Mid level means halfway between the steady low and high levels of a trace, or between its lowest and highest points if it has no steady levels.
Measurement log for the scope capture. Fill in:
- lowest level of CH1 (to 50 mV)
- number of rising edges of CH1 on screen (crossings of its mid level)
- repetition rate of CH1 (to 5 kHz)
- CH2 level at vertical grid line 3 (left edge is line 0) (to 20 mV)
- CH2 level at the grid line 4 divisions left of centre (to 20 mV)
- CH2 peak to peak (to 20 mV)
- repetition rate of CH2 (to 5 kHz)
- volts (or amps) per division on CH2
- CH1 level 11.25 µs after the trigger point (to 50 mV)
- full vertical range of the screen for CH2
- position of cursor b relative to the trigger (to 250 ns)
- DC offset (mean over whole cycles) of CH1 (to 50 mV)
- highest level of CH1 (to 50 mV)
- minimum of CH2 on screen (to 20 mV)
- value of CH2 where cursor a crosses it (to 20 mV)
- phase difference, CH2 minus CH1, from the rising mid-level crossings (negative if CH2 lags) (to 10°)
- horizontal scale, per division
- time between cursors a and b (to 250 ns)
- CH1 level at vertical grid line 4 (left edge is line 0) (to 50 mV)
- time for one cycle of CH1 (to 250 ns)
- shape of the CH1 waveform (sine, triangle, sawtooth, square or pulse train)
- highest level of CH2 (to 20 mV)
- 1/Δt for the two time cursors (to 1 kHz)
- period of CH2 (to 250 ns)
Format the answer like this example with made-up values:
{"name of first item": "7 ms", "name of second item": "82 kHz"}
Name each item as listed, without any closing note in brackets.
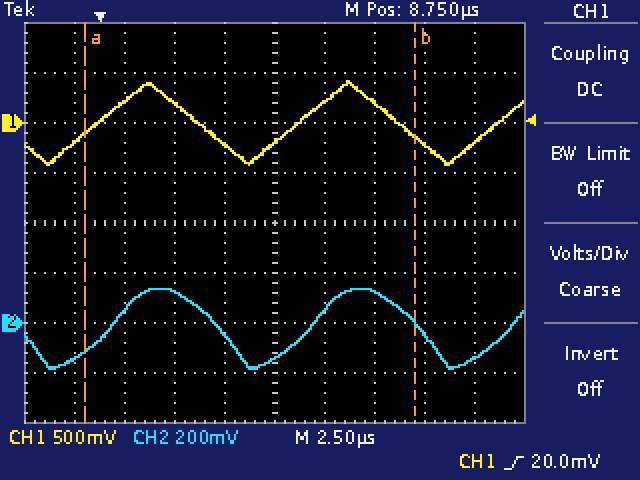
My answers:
{"lowest level of CH1": "-400 mV", "number of rising edges of CH1 on screen": "3", "repetition rate of CH1": "100 kHz", "CH2 level at vertical grid line 3 (left edge is line 0)": "120 mV", "CH2 level at the grid line 4 divisions left of centre": "-140 mV", "CH2 peak to peak": "320 mV", "repetition rate of CH2": "100 kHz", "volts (or amps) per division on CH2": "200 mV", "CH1 level 11.25 µs after the trigger point": "200 mV", "full vertical range of the screen for CH2": "1.6 V", "position of cursor b relative to the trigger": "+15.75 µs", "DC offset (mean over whole cycles) of CH1": "0 mV", "highest level of CH1": "400 mV", "minimum of CH2 on screen": "-180 mV", "value of CH2 where cursor a crosses it": "-120 mV", "phase difference, CH2 minus CH1, from the rising mid-level crossings (negative if CH2 lags)": "-20°", "horizontal scale, per division": "2.5 µs", "time between cursors a and b": "16.50 µs", "CH1 level at vertical grid line 4 (left edge is line 0)": "-200 mV", "time for one cycle of CH1": "10.00 µs", "shape of the CH1 waveform": "triangle", "highest level of CH2": "140 mV", "1/Δt for the two time cursors": "61 kHz", "period of CH2": "10.00 µs"}
